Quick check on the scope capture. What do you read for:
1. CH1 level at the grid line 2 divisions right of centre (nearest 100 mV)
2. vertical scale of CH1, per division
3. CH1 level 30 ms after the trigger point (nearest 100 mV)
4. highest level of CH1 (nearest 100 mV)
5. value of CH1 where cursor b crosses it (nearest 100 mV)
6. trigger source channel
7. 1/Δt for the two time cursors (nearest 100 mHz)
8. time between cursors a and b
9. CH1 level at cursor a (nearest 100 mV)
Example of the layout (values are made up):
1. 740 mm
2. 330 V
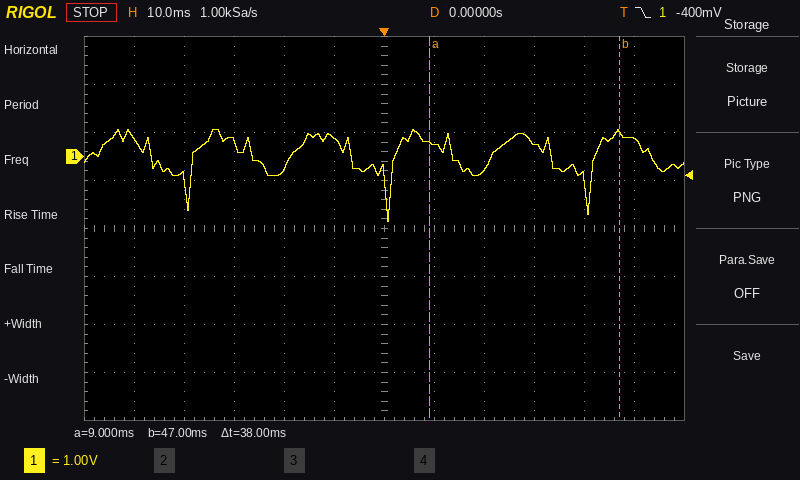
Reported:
1. -300 mV
2. 1 V
3. 300 mV
4. 600 mV
5. 500 mV
6. CH1
7. 26.3 Hz
8. 38 ms
9. 300 mV
